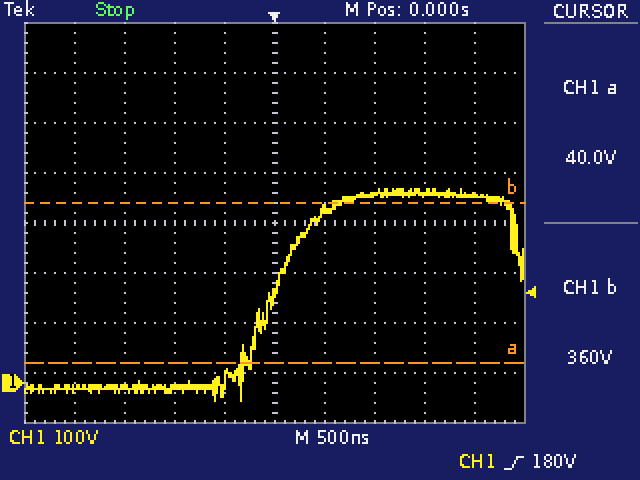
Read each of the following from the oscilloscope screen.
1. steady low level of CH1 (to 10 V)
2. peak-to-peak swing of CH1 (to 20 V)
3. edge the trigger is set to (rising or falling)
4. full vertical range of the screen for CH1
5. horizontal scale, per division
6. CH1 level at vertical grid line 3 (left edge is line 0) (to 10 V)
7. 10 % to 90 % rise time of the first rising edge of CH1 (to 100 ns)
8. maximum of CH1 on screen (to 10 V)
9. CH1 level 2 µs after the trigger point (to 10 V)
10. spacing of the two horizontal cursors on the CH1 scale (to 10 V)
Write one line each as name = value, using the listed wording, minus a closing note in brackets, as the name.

steady low level of CH1 = -10 V
peak-to-peak swing of CH1 = 420 V
edge the trigger is set to = rising
full vertical range of the screen for CH1 = 800 V
horizontal scale, per division = 500 ns
CH1 level at vertical grid line 3 (left edge is line 0) = -10 V
10 % to 90 % rise time of the first rising edge of CH1 = 800 ns
maximum of CH1 on screen = 390 V
CH1 level 2 µs after the trigger point = 380 V
spacing of the two horizontal cursors on the CH1 scale = 320 V
